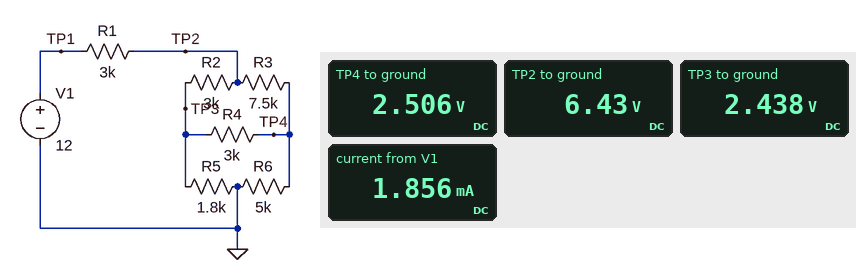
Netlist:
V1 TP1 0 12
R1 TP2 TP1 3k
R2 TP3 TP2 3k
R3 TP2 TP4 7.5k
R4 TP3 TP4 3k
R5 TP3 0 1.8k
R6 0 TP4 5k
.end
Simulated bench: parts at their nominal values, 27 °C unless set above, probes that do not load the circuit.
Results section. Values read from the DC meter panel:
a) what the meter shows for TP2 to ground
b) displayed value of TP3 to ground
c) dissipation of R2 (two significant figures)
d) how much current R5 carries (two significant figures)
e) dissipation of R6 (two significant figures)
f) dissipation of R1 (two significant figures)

6.43 V
2.438 V
5.3 mW
1.4 mA
1.3 mW
10 mW
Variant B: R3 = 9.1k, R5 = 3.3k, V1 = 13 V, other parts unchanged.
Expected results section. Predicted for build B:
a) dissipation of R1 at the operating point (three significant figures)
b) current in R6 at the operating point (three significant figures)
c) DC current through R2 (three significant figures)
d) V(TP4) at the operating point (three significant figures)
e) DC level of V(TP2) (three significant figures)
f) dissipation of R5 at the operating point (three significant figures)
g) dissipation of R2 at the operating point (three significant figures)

9.55 mW
649 µA
1.30 mA
3.25 V
7.65 V
4.25 mW
5.08 mW
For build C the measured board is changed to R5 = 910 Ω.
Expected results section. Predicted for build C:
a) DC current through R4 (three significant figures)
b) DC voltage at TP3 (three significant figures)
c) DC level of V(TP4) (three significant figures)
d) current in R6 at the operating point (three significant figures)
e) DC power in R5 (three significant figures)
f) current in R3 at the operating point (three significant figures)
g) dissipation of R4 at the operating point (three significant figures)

148 µA
1.49 V
1.93 V
386 µA
2.43 mW
535 µA
66.0 µW
